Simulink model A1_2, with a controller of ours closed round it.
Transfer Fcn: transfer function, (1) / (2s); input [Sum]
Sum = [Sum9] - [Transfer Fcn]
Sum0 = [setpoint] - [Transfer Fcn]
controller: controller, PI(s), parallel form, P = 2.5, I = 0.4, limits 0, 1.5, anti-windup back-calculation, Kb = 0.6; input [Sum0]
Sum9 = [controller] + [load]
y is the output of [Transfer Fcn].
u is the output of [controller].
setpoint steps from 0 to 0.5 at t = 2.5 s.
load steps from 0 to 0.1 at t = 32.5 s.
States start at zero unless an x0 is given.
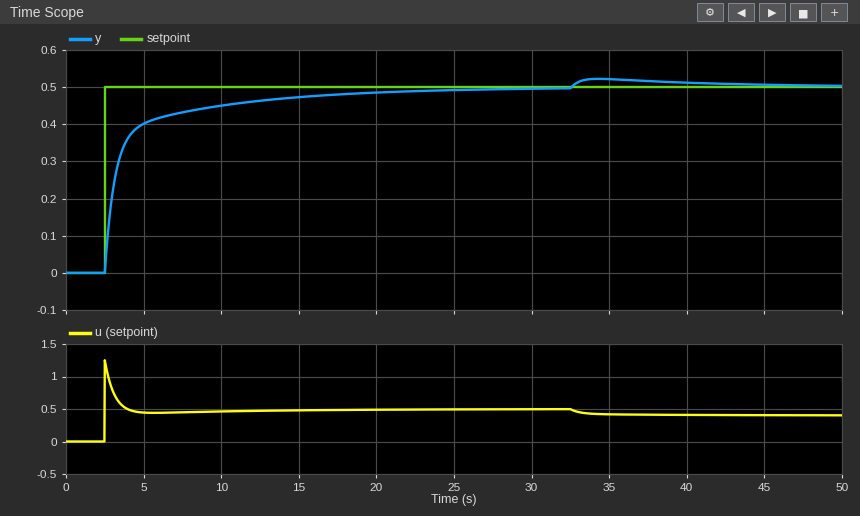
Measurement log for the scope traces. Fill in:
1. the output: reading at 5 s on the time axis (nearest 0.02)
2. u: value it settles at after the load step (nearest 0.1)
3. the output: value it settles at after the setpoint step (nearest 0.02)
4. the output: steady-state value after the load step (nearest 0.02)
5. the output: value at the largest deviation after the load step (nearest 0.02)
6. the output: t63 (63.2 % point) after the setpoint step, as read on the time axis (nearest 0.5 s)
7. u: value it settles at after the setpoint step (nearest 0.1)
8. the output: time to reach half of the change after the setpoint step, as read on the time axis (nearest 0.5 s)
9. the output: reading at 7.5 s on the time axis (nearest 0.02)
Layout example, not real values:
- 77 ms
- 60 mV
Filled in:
- 0.40
- 0.4
- 0.50
- 0.50
- 0.52
- 3.5 s
- 0.5
- 3.0 s
- 0.44
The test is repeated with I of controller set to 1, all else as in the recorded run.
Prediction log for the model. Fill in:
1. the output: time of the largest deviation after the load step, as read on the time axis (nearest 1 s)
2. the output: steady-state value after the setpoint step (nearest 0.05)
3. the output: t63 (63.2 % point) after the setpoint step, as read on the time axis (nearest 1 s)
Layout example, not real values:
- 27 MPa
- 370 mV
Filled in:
- 34 s
- 0.50
- 3 s
